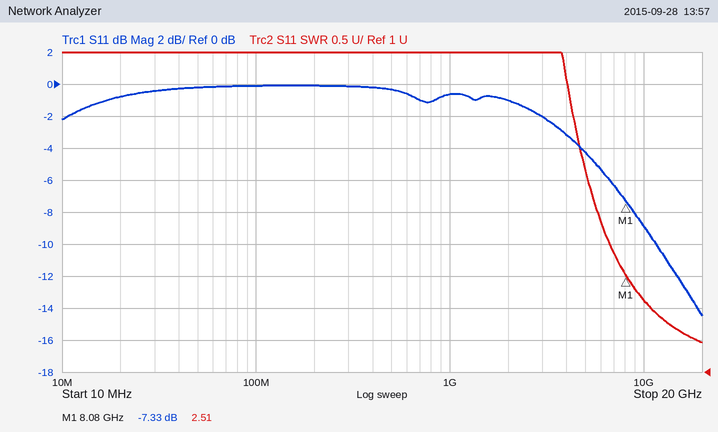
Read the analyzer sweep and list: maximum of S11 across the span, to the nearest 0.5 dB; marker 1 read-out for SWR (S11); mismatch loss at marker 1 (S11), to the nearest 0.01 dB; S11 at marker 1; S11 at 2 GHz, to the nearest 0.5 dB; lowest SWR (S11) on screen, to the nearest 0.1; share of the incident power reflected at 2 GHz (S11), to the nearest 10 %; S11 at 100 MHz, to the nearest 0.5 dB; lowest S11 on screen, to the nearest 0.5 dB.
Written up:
0.0 dB
2.51
0.89 dB
-7.33 dB
-1.0 dB
1.5
80 %
0.0 dB
-14.5 dB
